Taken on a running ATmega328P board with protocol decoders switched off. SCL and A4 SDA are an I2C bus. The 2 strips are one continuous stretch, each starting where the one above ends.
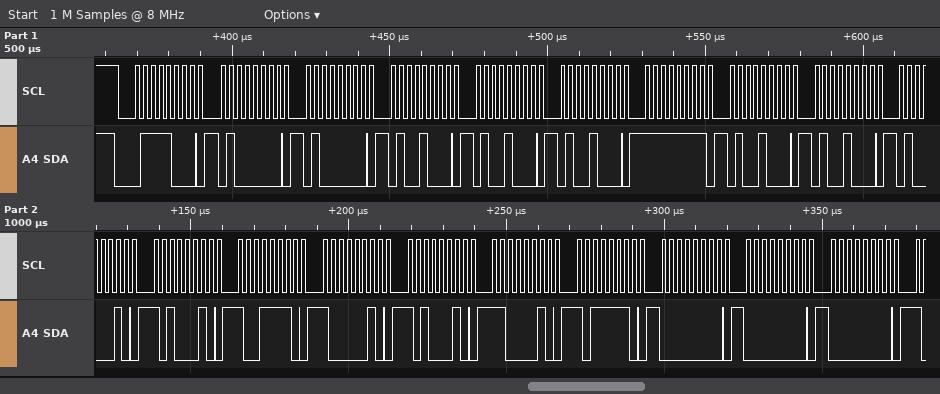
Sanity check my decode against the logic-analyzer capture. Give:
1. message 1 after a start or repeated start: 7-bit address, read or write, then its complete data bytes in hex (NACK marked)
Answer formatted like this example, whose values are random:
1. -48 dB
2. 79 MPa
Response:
1. 0x3C write: 40 40 48 48 48 FF 48 48 42 A2 9E 82 A2 C2 BE 00 00 00
